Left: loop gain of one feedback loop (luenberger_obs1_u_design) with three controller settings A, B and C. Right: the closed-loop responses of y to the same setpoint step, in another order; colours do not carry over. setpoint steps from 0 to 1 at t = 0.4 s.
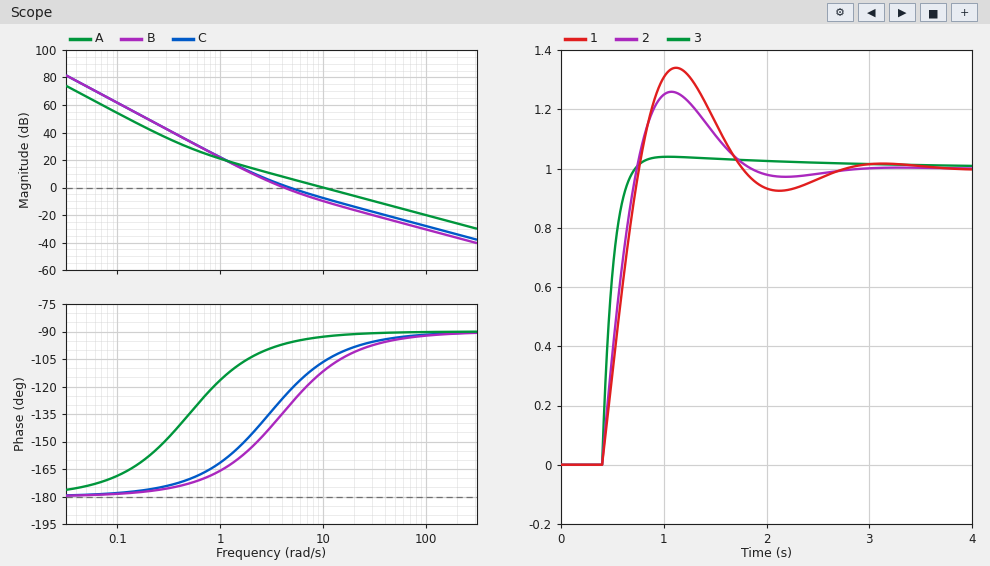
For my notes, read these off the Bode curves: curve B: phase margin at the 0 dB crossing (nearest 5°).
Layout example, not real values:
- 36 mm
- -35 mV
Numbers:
- 45°
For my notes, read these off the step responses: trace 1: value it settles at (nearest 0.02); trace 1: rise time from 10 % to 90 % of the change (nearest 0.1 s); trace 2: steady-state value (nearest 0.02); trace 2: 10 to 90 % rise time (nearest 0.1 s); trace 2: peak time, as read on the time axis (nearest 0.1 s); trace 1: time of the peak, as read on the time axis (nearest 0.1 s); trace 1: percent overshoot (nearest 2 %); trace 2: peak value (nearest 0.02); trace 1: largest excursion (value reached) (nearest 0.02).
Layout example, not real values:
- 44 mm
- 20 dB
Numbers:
- 1.00
- 0.3 s
- 1.00
- 0.3 s
- 1.1 s
- 1.1 s
- 34 %
- 1.26
- 1.34
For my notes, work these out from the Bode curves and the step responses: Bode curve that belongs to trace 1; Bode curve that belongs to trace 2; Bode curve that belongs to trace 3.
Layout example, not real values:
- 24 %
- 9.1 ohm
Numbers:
- B
- C
- A
